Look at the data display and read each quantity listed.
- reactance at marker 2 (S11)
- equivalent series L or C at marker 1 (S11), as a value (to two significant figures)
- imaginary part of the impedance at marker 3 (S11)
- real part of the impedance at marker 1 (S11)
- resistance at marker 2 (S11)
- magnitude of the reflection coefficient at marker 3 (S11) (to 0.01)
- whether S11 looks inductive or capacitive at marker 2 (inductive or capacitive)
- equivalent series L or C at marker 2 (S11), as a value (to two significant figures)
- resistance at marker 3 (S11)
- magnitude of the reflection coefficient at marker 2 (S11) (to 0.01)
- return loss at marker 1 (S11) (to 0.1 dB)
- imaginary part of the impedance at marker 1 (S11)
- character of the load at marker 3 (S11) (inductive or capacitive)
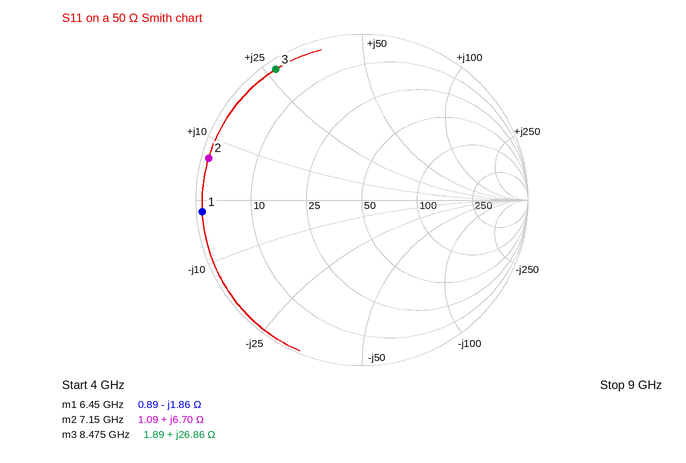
+6.70 Ω
13 pF
+26.86 Ω
0.89 Ω
1.09 Ω
0.94
inductive
150 pH
1.89 Ω
0.96
0.3 dB
-1.86 Ω
inductive
